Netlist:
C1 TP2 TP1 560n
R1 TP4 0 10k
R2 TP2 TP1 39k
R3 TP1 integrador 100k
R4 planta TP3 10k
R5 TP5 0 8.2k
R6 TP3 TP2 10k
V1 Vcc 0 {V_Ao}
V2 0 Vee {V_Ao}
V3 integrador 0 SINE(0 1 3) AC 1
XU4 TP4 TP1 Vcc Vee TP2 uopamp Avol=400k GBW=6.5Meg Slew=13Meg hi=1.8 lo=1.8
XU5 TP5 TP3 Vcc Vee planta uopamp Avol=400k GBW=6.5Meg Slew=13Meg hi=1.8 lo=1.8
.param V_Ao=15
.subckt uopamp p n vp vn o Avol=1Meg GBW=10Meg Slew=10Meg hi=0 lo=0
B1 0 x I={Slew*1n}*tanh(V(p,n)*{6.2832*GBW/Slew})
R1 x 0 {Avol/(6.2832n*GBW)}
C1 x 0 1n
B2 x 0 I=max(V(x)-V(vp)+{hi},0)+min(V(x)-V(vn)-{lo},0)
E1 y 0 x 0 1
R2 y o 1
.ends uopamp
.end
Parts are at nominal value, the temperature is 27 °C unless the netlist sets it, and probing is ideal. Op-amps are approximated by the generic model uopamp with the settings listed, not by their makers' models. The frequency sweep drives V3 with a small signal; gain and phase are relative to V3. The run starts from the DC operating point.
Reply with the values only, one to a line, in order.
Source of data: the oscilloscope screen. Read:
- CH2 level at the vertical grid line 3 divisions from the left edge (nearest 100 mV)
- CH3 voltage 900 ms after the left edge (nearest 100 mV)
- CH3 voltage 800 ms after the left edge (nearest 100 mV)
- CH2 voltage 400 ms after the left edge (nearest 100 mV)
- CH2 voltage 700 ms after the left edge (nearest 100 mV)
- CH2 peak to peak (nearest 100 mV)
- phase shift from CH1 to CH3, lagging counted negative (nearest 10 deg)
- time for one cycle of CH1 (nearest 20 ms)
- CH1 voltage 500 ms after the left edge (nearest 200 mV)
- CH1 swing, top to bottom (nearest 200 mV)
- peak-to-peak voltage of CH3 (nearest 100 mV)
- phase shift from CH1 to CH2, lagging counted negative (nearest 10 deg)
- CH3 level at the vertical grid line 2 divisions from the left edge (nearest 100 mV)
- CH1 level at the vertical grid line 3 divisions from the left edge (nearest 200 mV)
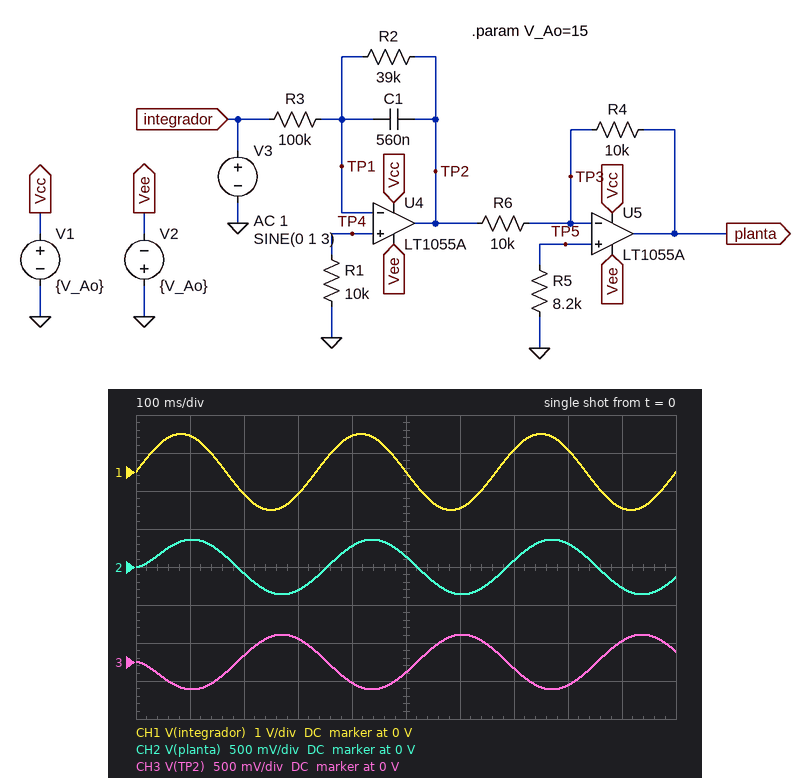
-300 mV
300 mV
-300 mV
300 mV
100 mV
700 mV
160 deg
340 ms
0 V
2.0 V
700 mV
-20 deg
100 mV
-600 mV
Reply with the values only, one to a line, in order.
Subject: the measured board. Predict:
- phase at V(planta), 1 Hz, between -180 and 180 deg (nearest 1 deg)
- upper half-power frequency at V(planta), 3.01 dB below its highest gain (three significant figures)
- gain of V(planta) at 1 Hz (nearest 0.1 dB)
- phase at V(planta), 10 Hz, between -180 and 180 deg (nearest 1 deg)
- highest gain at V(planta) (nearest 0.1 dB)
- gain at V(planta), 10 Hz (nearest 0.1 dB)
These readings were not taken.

-8 deg
7.29 Hz
-8.3 dB
-54 deg
-8.2 dB
-12.8 dB
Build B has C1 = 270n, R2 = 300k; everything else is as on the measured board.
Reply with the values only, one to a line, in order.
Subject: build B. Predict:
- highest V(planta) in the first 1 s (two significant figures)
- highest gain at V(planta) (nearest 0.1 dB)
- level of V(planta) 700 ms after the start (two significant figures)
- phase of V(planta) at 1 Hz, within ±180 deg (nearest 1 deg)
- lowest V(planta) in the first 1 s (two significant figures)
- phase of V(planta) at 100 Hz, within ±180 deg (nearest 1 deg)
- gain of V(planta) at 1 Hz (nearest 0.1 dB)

1.9 V
9.5 dB
-580 mV
-27 deg
-1.6 V
-89 deg
8.5 dB
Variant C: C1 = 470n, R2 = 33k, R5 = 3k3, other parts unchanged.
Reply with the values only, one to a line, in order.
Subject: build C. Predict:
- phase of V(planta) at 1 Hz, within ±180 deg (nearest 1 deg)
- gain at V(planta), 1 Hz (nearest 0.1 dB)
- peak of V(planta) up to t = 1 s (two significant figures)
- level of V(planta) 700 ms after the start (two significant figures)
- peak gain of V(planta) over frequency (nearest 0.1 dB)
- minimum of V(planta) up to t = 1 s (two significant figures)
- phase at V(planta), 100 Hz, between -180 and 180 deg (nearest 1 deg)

-6 deg
-9.7 dB
320 mV
110 mV
-9.6 dB
-320 mV
-84 deg
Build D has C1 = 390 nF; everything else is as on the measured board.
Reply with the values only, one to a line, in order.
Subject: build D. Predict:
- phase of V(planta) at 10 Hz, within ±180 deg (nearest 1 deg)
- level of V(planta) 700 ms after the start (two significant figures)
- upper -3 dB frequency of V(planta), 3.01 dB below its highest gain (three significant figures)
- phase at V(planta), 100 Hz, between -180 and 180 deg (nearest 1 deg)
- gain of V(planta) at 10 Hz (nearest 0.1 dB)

-44 deg
130 mV
10.5 Hz
-84 deg
-11.0 dB
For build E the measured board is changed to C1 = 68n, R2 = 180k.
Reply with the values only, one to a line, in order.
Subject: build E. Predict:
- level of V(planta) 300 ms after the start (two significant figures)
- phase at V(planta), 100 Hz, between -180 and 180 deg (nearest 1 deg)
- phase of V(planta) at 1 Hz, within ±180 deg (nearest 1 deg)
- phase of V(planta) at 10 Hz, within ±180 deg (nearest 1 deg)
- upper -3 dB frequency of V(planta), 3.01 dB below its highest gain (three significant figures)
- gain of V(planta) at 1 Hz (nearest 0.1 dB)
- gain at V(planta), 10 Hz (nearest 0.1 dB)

-1.3 V
-83 deg
-4 deg
-38 deg
13.0 Hz
5.1 dB
3.1 dB
